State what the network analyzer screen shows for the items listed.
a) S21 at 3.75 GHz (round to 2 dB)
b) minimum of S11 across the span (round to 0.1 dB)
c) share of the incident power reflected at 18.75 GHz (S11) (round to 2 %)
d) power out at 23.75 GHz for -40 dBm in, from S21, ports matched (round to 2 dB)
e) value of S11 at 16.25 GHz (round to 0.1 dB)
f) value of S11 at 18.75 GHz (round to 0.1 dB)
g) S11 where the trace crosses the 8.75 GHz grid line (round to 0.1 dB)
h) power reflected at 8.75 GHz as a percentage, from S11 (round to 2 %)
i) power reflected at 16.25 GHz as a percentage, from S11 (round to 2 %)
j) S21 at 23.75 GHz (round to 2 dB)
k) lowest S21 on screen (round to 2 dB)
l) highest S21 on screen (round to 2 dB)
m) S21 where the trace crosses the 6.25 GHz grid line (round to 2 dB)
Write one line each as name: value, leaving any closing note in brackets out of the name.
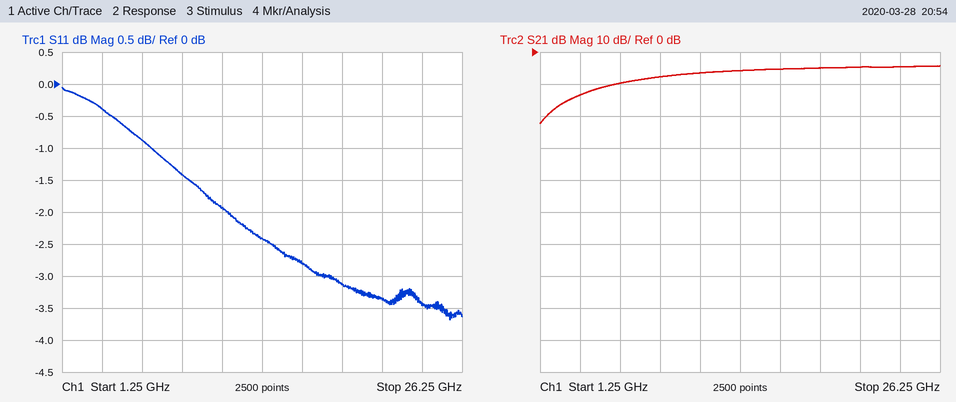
S21 at 3.75 GHz: -14 dB
minimum of S11 across the span: -3.7 dB
share of the incident power reflected at 18.75 GHz (S11): 48 %
power out at 23.75 GHz for -40 dBm in, from S21, ports matched: -44 dBm
value of S11 at 16.25 GHz: -2.8 dB
value of S11 at 18.75 GHz: -3.1 dB
S11 where the trace crosses the 8.75 GHz grid line: -1.4 dB
power reflected at 8.75 GHz as a percentage, from S11: 72 %
power reflected at 16.25 GHz as a percentage, from S11: 52 %
S21 at 23.75 GHz: -4 dB
lowest S21 on screen: -22 dB
highest S21 on screen: -4 dB
S21 where the trace crosses the 6.25 GHz grid line: -10 dB
